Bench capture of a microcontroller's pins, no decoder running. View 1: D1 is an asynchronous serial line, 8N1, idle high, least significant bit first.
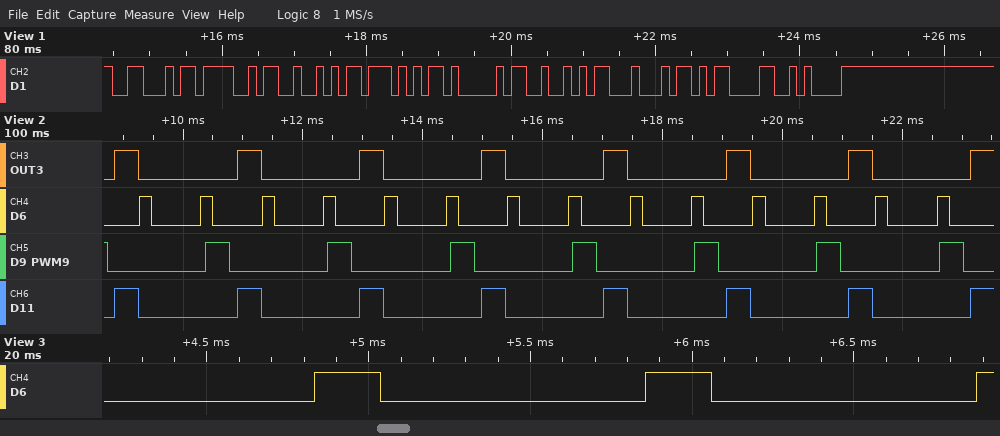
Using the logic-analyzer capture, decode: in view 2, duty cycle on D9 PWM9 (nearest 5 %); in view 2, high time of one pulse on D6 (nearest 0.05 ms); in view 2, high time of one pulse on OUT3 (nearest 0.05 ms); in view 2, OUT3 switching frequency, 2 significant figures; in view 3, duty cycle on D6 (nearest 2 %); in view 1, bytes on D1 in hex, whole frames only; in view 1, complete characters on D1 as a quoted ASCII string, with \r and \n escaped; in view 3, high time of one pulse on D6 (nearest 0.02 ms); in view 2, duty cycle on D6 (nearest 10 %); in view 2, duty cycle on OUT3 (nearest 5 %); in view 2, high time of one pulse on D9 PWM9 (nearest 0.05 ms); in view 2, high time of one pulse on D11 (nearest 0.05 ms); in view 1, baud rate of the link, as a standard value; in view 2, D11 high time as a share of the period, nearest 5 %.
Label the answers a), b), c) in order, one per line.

a) 20 %
b) 0.20 ms
c) 0.40 ms
d) 490 Hz
e) 20 %
f) 0x46 0x4F 0x52 0x57 0x41 0x52 0x44 0x0D 0x0A
g) "FORWARD\r\n"
h) 0.20 ms
i) 20 %
j) 20 %
k) 0.40 ms
l) 0.40 ms
m) 9600 baud
n) 20 %
